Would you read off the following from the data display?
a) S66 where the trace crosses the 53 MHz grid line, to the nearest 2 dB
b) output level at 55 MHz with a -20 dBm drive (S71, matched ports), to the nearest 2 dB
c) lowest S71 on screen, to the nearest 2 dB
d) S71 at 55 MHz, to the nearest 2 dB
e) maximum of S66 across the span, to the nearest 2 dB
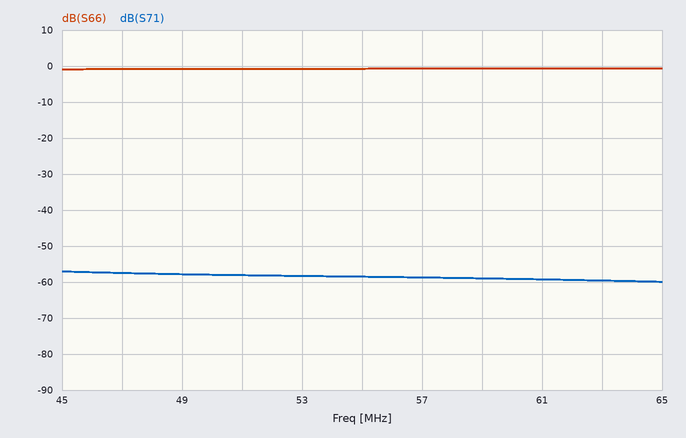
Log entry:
0 dB
-78 dBm
-60 dB
-58 dB
0 dB
